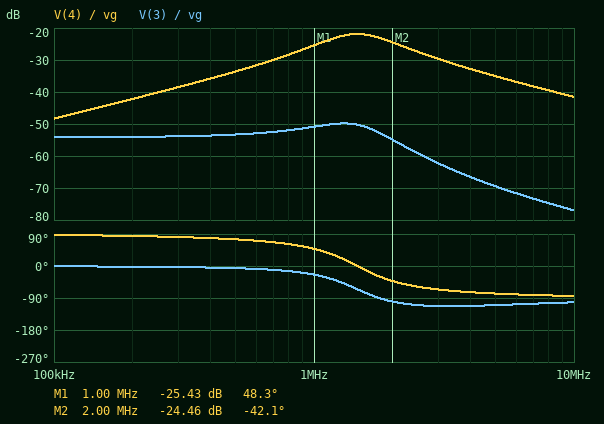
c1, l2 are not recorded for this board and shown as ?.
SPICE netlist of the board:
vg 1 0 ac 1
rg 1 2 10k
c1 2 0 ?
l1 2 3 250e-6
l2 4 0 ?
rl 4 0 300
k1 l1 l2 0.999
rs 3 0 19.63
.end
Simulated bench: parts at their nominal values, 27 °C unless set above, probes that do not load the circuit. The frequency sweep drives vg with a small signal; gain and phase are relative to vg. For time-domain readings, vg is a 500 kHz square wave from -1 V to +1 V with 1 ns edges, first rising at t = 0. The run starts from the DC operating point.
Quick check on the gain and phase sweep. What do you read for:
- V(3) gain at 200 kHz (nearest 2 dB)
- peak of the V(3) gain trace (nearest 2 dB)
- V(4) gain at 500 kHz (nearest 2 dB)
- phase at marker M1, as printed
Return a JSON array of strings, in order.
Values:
["-54 dB", "-50 dB", "-34 dB", "48.3 deg"]
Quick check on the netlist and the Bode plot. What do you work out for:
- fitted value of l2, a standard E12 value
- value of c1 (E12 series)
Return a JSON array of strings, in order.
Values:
["15 µH", "47 pF"]
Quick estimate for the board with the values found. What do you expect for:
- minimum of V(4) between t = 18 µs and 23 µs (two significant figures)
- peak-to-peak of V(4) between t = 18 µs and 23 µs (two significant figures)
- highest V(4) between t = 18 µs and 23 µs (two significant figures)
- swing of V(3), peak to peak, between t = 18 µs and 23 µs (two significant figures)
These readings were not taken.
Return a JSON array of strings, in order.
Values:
["-73 mV", "150 mV", "73 mV", "6.7 mV"]
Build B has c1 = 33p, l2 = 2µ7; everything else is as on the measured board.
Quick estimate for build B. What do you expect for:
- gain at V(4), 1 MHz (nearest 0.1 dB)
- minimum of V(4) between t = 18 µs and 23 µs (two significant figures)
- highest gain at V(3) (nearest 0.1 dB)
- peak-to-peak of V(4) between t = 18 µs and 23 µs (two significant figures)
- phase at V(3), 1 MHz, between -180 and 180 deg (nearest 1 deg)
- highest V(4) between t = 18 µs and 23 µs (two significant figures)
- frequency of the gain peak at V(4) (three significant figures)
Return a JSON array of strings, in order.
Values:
["-32.8 dB", "-45 mV", "-45.6 dB", "91 mV", "-15 deg", "45 mV", "1.75 MHz"]
